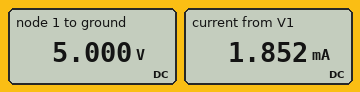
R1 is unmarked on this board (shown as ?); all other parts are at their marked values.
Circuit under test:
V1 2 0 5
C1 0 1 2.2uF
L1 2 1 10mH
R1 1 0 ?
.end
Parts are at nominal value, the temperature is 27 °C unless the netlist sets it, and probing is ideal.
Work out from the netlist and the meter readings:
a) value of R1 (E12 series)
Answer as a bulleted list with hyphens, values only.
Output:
- 2.7 kΩ
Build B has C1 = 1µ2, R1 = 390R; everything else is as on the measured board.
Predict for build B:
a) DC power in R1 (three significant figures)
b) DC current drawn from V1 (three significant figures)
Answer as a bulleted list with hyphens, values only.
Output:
- 64.1 mW
- 12.8 mA
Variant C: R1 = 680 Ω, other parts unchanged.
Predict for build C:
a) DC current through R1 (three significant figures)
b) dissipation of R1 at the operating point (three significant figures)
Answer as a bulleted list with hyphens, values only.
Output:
- 7.35 mA
- 36.8 mW
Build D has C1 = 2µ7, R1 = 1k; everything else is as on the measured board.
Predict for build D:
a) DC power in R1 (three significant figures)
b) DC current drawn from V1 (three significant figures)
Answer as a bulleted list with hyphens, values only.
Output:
- 25.0 mW
- 5.00 mA
